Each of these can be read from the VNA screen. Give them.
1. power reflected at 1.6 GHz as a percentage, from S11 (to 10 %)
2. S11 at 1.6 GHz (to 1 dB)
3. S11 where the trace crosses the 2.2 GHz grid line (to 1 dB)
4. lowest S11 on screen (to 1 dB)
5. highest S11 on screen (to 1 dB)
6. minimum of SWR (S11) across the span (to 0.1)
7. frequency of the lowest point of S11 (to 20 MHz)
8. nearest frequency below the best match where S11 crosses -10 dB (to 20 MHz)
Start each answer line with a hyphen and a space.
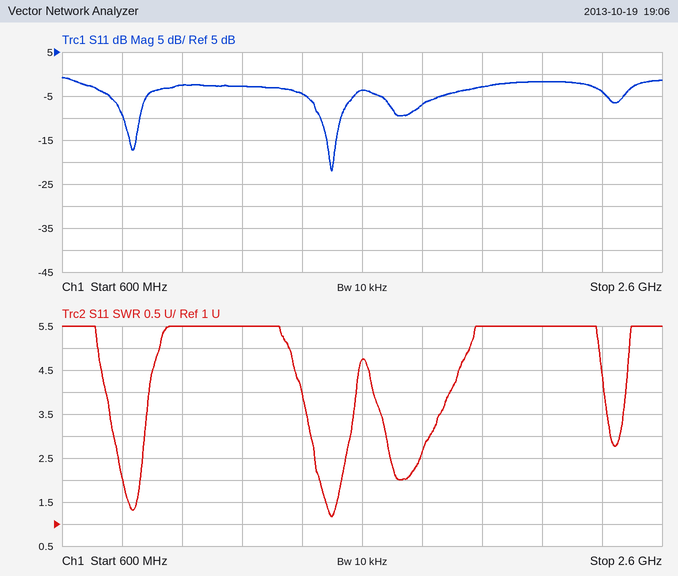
- 40 %
- -4 dB
- -2 dB
- -22 dB
- -1 dB
- 1.2
- 1.50 GHz
- 1.46 GHz
